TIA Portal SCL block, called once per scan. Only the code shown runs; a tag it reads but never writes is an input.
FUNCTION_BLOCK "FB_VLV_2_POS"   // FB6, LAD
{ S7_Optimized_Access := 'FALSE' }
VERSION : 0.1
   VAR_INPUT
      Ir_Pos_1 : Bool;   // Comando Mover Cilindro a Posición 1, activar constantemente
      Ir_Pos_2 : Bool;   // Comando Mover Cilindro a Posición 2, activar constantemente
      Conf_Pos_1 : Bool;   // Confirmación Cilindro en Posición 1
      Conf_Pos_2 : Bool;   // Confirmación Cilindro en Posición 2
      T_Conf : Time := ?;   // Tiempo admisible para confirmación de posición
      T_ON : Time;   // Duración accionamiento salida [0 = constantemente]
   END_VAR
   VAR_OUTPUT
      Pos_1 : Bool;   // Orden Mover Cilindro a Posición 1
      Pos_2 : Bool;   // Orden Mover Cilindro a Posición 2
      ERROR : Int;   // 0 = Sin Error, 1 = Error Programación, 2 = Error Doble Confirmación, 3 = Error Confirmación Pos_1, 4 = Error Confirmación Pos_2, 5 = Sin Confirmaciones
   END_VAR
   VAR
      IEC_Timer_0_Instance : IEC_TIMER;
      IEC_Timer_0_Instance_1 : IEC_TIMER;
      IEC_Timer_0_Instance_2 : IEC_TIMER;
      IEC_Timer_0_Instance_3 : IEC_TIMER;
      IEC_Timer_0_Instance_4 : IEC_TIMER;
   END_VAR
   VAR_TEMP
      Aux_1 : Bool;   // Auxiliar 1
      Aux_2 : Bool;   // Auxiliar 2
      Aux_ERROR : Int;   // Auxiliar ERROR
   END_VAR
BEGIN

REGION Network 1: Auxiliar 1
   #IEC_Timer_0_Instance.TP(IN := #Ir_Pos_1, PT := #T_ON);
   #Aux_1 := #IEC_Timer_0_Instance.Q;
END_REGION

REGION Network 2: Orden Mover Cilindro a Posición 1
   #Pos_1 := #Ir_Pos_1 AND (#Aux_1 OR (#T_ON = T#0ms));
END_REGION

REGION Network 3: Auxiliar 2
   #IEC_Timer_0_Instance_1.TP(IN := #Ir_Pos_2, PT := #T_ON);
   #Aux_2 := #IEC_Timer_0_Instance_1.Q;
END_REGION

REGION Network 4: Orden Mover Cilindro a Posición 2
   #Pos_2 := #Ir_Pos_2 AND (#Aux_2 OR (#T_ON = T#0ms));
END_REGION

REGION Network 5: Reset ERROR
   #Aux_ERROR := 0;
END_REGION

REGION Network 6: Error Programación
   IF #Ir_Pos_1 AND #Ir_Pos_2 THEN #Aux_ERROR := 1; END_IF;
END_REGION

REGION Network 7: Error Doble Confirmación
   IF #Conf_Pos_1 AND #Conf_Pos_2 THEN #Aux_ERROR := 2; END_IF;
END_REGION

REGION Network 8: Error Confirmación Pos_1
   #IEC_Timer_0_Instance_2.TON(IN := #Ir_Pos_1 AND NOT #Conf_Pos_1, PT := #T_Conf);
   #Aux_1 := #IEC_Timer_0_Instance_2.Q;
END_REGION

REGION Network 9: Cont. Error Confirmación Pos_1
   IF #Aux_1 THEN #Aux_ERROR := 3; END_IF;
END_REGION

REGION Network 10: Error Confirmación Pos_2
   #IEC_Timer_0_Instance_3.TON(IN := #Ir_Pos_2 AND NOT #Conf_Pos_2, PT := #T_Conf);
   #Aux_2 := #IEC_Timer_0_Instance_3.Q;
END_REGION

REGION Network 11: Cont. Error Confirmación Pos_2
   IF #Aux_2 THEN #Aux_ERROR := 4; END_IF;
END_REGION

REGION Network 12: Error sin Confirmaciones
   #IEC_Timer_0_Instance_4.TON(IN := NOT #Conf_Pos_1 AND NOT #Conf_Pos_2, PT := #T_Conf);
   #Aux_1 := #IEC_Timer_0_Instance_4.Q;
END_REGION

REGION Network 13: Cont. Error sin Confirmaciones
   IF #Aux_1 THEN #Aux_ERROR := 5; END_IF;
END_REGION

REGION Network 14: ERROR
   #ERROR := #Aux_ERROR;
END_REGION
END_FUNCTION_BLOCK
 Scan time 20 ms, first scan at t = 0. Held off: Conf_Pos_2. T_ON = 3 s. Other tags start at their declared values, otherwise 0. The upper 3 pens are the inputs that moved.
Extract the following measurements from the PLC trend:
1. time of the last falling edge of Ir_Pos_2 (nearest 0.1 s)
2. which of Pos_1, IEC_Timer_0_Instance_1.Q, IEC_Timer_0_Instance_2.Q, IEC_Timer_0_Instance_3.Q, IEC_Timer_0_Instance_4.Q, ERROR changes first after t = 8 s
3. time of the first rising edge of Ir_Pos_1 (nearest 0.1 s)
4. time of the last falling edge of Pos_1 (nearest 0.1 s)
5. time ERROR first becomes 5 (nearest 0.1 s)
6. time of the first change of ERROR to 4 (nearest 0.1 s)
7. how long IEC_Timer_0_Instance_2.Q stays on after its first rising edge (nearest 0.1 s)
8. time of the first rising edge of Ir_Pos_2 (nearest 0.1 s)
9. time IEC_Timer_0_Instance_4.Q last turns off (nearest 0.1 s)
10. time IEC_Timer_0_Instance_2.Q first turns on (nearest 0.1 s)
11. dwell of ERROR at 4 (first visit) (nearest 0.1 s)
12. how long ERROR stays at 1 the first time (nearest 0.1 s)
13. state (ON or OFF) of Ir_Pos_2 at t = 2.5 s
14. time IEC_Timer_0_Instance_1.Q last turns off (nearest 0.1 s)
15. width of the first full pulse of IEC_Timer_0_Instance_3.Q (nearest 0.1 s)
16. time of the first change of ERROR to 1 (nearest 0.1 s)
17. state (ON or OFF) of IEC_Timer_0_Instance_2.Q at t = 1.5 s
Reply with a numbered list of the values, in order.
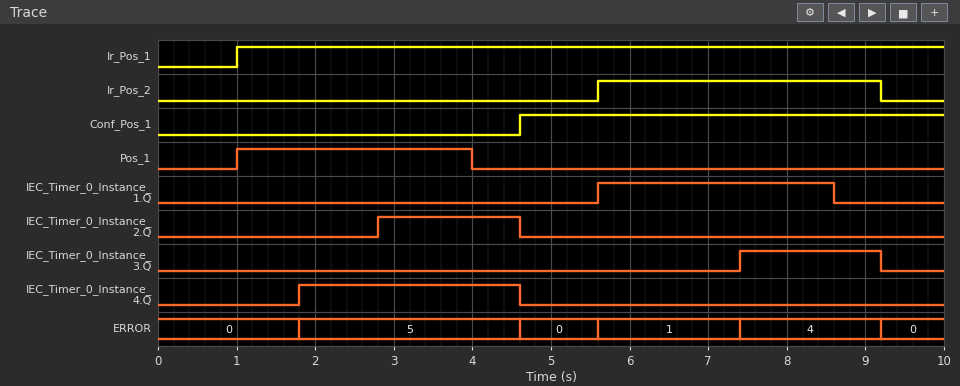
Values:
1. 9.2 s
2. IEC_Timer_0_Instance_1.Q
3. 1.0 s
4. 4.0 s
5. 1.8 s
6. 7.4 s
7. 1.8 s
8. 5.6 s
9. 4.6 s
10. 2.8 s
11. 1.8 s
12. 1.8 s
13. OFF
14. 8.6 s
15. 1.8 s
16. 5.6 s
17. OFF
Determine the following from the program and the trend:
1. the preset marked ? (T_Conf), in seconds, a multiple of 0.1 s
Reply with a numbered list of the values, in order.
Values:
1. 1.8 s
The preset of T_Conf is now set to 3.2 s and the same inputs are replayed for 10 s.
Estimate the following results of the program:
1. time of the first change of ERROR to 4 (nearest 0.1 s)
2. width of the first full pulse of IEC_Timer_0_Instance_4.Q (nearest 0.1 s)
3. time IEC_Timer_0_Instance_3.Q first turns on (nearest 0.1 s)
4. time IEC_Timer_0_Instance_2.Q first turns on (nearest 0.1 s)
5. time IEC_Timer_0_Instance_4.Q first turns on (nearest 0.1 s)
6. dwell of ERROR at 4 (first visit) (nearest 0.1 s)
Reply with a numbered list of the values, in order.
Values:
1. 8.8 s
2. 1.4 s
3. 8.8 s
4. 4.2 s
5. 3.2 s
6. 0.4 s
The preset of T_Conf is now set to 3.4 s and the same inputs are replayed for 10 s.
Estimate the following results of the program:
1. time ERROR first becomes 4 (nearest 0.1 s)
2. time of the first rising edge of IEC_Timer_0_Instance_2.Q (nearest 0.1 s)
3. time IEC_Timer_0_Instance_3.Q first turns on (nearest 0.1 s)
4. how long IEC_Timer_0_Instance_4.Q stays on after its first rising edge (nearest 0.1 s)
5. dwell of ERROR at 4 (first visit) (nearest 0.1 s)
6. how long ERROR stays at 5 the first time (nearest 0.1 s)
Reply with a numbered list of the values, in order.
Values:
1. 9.0 s
2. 4.4 s
3. 9.0 s
4. 1.2 s
5. 0.2 s
6. 1.2 s
